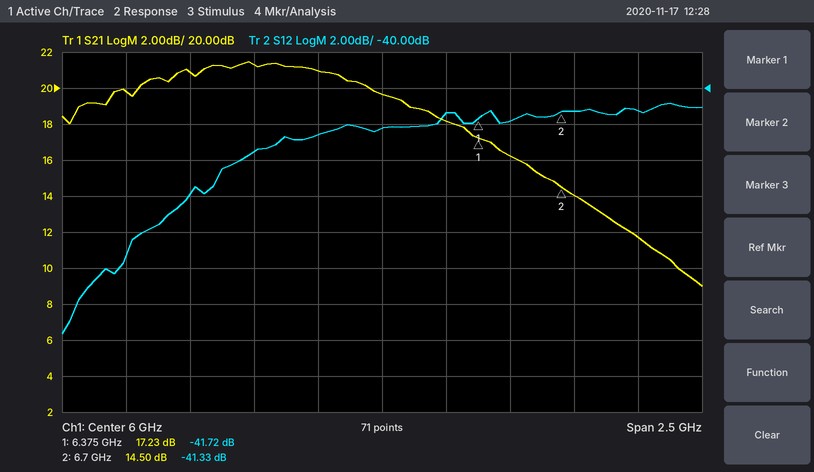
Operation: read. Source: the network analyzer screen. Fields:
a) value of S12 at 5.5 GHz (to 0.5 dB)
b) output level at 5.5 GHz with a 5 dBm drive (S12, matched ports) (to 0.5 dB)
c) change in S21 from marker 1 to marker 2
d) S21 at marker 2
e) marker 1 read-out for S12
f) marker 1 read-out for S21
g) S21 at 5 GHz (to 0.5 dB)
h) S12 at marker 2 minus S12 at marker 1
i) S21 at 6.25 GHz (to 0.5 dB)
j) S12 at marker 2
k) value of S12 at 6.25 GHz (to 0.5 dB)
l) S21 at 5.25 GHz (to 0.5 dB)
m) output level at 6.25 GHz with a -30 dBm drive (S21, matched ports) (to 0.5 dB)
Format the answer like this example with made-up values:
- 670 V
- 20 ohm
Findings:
- -43.5 dB
- -38.5 dBm
- -2.73 dB
- 14.50 dB
- -41.72 dB
- 17.23 dB
- 20.0 dB
- 0.39 dB
- 18.0 dB
- -41.33 dB
- -41.5 dB
- 21.0 dB
- -12.0 dBm
